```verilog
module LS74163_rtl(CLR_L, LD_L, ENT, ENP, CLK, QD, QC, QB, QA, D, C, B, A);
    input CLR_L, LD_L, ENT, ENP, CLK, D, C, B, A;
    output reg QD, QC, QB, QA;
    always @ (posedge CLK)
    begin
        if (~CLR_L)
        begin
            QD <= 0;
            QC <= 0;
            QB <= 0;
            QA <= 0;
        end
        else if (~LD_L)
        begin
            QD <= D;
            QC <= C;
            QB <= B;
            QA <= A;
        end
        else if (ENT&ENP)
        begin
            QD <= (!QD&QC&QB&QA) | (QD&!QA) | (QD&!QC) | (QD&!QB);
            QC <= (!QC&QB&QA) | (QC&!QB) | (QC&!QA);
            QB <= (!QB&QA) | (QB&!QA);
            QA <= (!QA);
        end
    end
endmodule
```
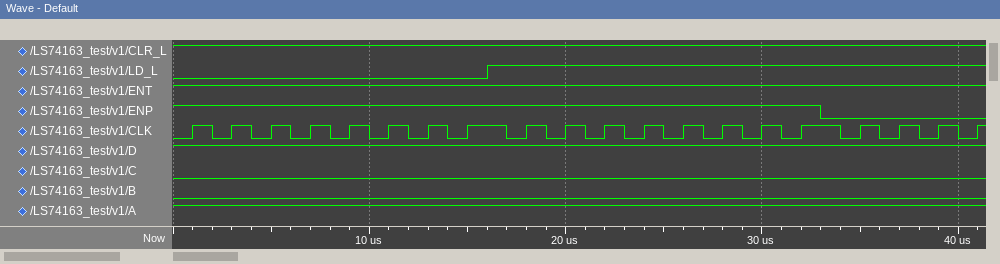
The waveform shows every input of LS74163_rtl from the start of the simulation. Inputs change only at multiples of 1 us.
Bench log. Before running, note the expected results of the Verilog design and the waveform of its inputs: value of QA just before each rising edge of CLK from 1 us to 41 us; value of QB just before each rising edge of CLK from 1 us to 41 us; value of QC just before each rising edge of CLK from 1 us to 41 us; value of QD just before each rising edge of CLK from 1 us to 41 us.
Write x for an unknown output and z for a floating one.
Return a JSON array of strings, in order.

["x 1 1 1 1 1 1 1 1 0 1 0 1 0 1 0 1 1 1 1", "x 0 0 0 0 0 0 0 0 1 1 0 0 1 1 0 0 0 0 0", "x 0 0 0 0 0 0 0 0 0 0 1 1 1 1 0 0 0 0 0", "x 1 1 1 1 1 1 1 1 1 1 1 1 1 1 0 0 0 0 0"]
